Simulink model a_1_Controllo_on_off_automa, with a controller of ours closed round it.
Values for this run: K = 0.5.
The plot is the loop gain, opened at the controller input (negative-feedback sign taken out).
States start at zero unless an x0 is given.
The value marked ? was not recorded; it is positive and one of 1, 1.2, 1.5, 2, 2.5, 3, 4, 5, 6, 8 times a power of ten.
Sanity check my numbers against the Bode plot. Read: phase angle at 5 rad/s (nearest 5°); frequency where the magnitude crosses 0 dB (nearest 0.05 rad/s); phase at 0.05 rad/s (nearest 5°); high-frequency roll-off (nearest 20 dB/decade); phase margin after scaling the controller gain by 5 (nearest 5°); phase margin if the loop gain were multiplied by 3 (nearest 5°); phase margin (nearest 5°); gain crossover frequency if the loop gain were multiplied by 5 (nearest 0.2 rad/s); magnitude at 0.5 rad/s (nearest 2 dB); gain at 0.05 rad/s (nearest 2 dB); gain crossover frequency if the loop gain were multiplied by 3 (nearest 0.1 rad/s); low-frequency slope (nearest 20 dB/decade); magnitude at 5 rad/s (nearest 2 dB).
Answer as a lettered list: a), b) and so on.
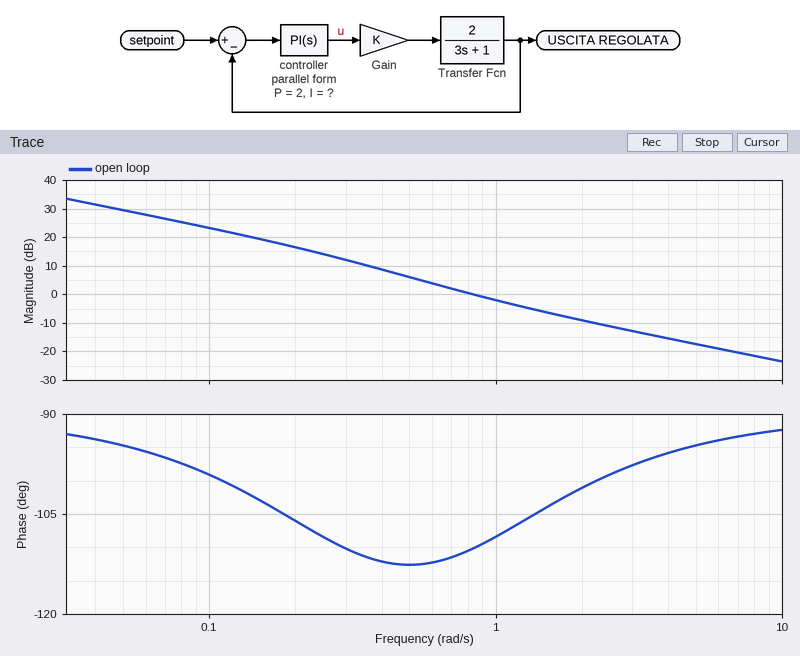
a) -95°
b) 0.85 rad/s
c) -95°
d) -20 dB/decade
e) 85°
f) 80°
g) 70°
h) 3.4 rad/s
i) 6 dB
j) 30 dB
k) 2.1 rad/s
l) -20 dB/decade
m) -18 dB
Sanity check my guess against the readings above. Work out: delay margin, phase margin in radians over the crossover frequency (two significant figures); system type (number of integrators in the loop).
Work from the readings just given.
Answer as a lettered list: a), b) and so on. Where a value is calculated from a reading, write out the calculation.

a) 70 × π / 180 / 0.85 = 1.4 s
b) 1
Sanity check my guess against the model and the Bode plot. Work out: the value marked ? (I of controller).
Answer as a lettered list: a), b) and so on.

a) 1.5
